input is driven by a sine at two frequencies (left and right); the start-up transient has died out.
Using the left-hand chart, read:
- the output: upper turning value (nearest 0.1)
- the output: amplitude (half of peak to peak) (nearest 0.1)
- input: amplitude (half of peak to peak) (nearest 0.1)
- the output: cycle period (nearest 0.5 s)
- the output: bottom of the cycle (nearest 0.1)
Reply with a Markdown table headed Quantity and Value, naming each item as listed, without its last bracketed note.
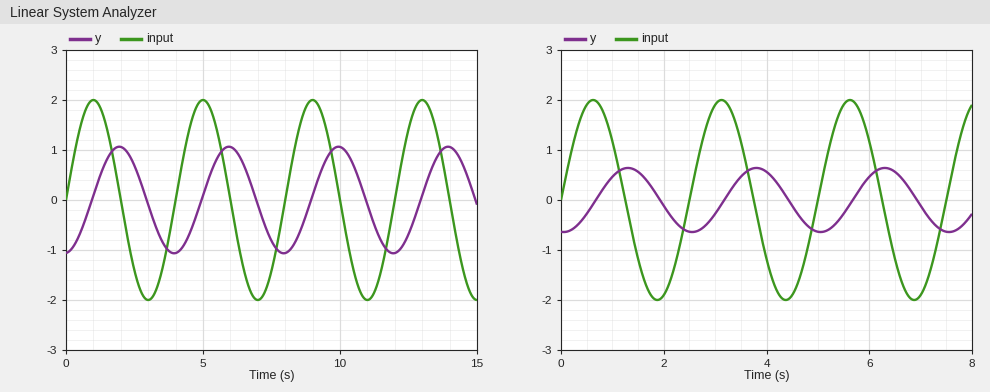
| Quantity | Value |
|---|---|
| the output: upper turning value | 1.1 |
| the output: amplitude (half of peak to peak) | 1.1 |
| input: amplitude (half of peak to peak) | 2.0 |
| the output: cycle period | 4.0 s |
| the output: bottom of the cycle | -1.1 |
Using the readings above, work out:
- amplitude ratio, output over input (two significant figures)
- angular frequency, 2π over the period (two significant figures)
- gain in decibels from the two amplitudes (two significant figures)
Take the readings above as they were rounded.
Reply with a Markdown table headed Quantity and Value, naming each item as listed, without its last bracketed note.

| Quantity | Value |
|---|---|
| amplitude ratio, output over input | 0.55 |
| angular frequency, 2π over the period | 1.6 rad/s |
| gain in decibels from the two amplitudes | -5.2 dB |
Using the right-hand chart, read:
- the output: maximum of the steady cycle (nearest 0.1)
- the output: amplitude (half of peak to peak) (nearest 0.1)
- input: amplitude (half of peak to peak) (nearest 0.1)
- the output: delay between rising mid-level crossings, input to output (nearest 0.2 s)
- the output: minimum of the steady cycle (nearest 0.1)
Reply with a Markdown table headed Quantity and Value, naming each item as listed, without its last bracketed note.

| Quantity | Value |
|---|---|
| the output: maximum of the steady cycle | 0.6 |
| the output: amplitude (half of peak to peak) | 0.6 |
| input: amplitude (half of peak to peak) | 2.0 |
| the output: delay between rising mid-level crossings, input to output | 0.6 s |
| the output: minimum of the steady cycle | -0.6 |
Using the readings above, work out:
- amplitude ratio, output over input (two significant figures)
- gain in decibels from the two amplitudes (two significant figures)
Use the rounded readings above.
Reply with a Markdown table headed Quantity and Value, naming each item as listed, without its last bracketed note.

| Quantity | Value |
|---|---|
| amplitude ratio, output over input | 0.30 |
| gain in decibels from the two amplitudes | -10 dB |
